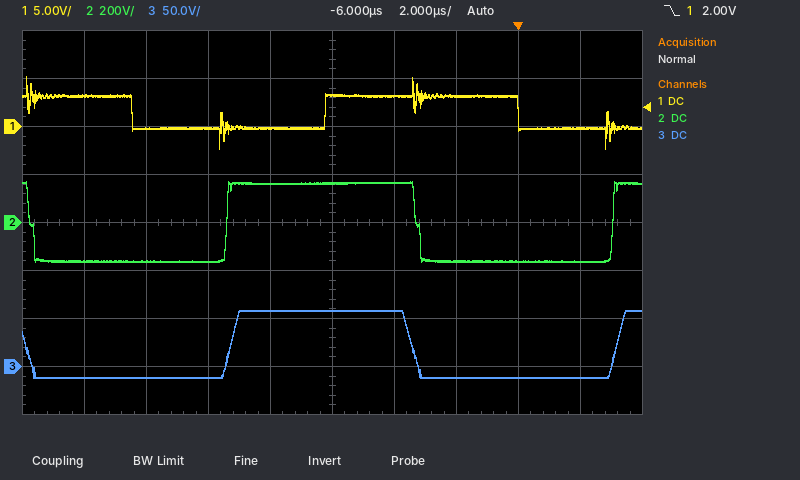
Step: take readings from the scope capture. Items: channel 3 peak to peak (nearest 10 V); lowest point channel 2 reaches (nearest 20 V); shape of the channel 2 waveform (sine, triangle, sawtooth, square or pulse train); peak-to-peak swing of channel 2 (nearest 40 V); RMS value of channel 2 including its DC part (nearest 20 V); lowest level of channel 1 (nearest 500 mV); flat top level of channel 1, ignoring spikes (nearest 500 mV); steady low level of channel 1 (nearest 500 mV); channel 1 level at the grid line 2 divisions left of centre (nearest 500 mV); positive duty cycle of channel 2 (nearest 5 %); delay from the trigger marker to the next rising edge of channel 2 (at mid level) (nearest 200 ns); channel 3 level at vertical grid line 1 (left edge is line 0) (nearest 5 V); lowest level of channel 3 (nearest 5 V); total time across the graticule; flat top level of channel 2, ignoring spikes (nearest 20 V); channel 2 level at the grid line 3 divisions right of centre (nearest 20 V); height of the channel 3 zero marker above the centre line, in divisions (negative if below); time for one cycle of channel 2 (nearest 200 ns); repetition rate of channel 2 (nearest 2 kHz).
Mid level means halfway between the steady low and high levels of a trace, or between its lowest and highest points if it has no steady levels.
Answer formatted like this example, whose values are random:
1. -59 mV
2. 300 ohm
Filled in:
1. 70 V
2. -160 V
3. square
4. 320 V
5. 160 V
6. -2.5 V
7. 3.0 V
8. 0.0 V
9. 0.0 V
10. 50 %
11. 3.0 µs
12. -10 V
13. -10 V
14. 20 µs
15. 160 V
16. -160 V
17. -3.0 div
18. 12.4 µs
19. 80 kHz
